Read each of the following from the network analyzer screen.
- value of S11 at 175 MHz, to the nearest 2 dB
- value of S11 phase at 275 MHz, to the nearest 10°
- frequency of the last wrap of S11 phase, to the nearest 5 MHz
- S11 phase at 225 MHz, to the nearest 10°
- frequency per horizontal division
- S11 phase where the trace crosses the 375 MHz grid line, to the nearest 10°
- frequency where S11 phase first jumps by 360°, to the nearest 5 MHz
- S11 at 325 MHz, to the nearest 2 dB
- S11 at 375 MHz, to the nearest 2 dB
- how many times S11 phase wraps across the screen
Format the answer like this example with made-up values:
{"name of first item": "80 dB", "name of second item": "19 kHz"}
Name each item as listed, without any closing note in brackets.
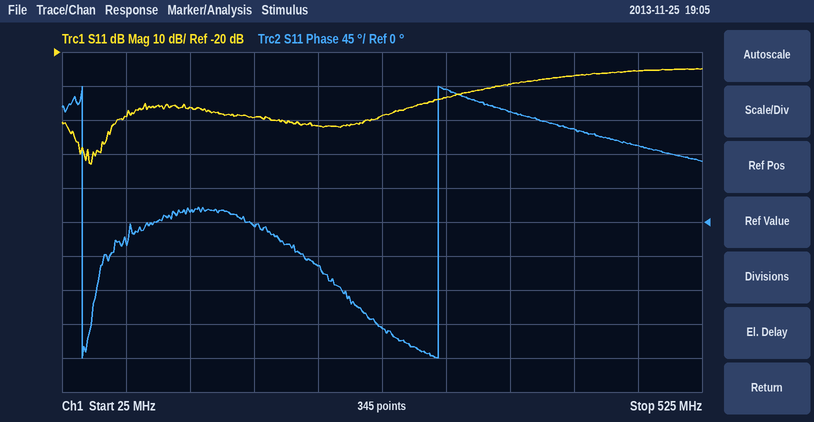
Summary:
{"value of S11 at 175 MHz, to the nearest 2 dB": "-40 dB", "value of S11 phase at 275 MHz, to the nearest 10°": "-140°", "frequency of the last wrap of S11 phase, to the nearest 5 MHz": "320 MHz", "S11 phase at 225 MHz, to the nearest 10°": "-60°", "frequency per horizontal division": "50 MHz", "S11 phase where the trace crosses the 375 MHz grid line, to the nearest 10°": "150°", "frequency where S11 phase first jumps by 360°, to the nearest 5 MHz": "40 MHz", "S11 at 325 MHz, to the nearest 2 dB": "-34 dB", "S11 at 375 MHz, to the nearest 2 dB": "-30 dB", "how many times S11 phase wraps across the screen": "2"}
